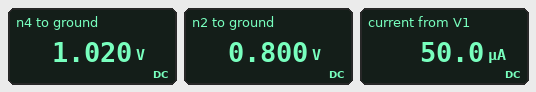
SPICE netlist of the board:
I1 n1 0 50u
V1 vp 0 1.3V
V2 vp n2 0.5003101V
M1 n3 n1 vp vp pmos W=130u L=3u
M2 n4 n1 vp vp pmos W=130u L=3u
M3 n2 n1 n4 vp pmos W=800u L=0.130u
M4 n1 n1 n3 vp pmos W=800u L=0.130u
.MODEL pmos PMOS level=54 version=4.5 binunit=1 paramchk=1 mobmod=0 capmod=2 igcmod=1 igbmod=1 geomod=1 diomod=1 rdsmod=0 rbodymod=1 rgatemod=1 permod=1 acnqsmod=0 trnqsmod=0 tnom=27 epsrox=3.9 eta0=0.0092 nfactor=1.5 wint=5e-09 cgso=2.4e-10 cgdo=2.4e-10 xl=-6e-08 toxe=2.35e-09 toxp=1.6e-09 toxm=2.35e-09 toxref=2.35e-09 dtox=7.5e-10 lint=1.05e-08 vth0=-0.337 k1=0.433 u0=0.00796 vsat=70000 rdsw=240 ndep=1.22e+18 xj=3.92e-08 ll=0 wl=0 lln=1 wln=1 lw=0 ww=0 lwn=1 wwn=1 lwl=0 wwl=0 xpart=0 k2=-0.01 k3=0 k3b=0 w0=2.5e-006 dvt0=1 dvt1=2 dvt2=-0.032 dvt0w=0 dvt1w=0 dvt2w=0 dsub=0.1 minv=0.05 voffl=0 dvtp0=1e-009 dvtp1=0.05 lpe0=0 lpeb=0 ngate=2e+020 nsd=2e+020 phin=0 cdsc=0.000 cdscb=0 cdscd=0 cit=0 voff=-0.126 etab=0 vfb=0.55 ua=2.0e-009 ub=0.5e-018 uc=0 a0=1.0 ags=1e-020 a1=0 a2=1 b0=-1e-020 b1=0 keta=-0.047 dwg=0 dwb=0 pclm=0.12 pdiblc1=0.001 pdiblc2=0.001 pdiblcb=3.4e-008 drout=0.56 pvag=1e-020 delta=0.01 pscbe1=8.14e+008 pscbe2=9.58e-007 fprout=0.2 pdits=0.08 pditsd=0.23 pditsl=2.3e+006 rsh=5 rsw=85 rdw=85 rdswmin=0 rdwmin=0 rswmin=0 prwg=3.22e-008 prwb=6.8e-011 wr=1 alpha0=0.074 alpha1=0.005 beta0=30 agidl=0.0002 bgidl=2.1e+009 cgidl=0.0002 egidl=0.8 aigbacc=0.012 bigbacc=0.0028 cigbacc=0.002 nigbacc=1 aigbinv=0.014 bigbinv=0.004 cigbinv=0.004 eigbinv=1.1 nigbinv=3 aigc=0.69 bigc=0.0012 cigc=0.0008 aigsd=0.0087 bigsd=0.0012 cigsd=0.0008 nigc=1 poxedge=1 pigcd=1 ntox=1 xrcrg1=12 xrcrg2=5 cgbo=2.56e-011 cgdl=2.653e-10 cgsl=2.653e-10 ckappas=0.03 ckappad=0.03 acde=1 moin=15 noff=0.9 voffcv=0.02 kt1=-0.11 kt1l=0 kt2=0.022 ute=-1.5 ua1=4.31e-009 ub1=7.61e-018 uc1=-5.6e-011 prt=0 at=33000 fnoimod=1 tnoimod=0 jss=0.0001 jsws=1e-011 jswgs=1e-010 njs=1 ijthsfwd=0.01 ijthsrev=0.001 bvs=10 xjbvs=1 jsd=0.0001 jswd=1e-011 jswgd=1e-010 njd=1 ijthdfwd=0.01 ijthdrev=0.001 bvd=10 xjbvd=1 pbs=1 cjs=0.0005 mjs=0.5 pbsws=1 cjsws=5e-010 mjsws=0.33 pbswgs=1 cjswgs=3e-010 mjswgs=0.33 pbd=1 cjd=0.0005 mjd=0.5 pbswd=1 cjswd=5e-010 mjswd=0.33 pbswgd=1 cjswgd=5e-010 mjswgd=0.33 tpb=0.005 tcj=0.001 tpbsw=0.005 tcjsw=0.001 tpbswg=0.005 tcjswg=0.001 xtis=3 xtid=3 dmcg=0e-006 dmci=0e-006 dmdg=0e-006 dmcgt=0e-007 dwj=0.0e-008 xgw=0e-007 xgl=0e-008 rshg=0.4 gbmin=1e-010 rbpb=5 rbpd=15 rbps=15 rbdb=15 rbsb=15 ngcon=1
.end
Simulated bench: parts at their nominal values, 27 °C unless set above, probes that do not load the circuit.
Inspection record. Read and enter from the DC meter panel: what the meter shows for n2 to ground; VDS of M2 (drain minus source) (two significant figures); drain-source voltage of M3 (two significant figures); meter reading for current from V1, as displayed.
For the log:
0.800 V
-280 mV
-220 mV
50.0 µA
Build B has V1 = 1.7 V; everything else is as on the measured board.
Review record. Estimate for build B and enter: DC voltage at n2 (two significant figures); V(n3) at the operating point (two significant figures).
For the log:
1.2 V
1.4 V
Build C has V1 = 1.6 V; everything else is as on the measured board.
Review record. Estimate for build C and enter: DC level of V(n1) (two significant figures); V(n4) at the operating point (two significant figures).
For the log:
1.1 V
1.3 V
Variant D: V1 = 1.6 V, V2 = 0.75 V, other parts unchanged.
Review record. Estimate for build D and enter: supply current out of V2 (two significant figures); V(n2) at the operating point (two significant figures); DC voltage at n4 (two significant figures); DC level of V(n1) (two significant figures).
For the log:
50 µA
850 mV
1.3 V
1.1 V
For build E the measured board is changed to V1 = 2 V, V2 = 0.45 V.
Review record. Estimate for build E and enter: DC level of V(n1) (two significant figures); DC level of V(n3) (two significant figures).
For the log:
1.5 V
1.7 V
